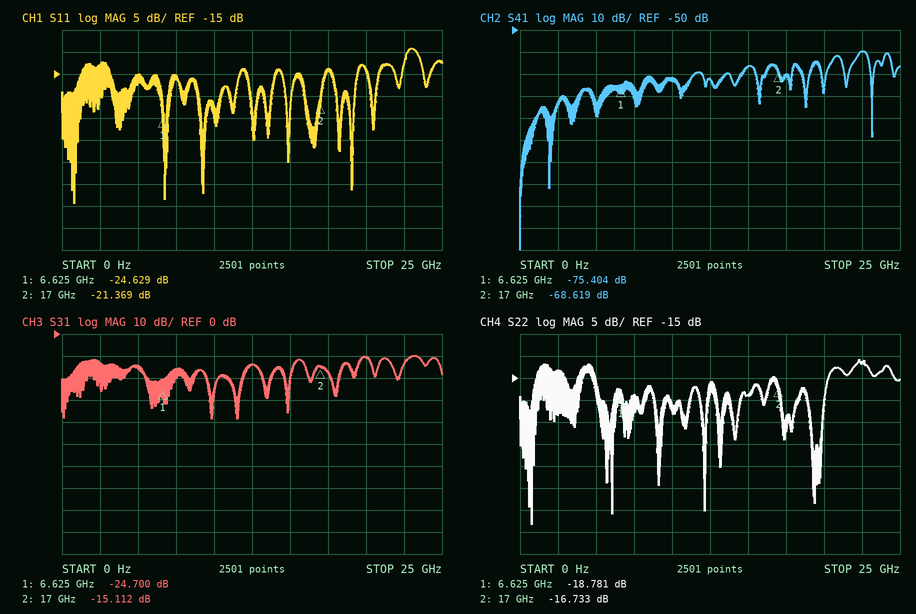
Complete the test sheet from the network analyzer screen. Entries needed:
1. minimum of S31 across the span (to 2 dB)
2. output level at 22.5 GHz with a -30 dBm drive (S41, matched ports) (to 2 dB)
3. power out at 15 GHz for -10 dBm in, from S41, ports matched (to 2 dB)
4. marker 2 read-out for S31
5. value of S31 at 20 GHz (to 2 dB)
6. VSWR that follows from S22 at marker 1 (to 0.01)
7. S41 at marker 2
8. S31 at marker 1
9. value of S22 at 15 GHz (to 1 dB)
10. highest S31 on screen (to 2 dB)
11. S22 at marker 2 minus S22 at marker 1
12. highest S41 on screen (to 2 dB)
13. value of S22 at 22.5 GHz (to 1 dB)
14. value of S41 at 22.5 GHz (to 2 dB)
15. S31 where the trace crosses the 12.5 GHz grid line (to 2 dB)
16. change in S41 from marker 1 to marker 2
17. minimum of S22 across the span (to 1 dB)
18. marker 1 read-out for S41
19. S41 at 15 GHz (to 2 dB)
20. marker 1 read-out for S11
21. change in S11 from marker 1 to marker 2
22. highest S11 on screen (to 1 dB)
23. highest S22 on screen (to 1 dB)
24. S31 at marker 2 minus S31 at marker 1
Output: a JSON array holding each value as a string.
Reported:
["-38 dB", "-90 dBm", "-76 dBm", "-15.112 dB", "-10 dB", "1.26", "-68.619 dB", "-24.700 dB", "-19 dB", "-10 dB", "2.048 dB", "-60 dB", "-11 dB", "-60 dB", "-14 dB", "6.785 dB", "-48 dB", "-75.404 dB", "-66 dB", "-24.629 dB", "3.260 dB", "-9 dB", "-11 dB", "9.588 dB"]
